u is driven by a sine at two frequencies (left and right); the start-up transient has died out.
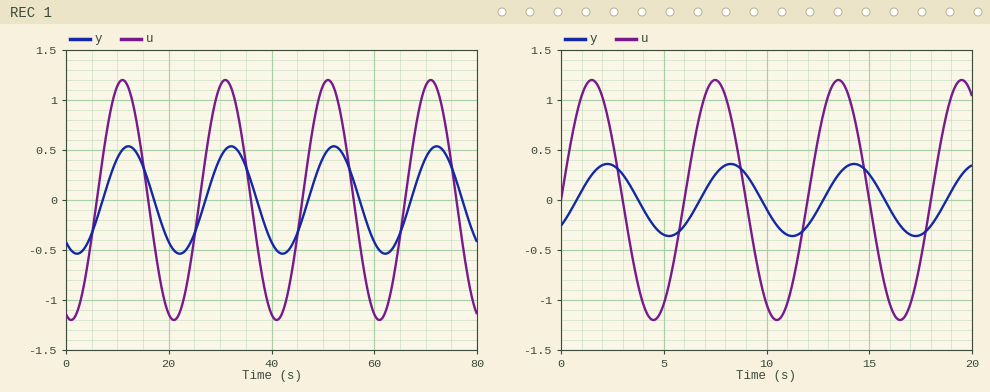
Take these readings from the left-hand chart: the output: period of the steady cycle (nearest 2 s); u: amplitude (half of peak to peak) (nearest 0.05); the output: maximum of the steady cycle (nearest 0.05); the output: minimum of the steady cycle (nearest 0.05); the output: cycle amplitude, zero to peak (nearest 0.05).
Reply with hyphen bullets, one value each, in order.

- 20 s
- 1.20
- 0.55
- -0.55
- 0.55
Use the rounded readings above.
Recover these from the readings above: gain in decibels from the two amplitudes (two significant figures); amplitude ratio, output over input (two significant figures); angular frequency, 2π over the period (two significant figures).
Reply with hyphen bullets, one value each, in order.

- -6.8 dB
- 0.46
- 0.31 rad/s
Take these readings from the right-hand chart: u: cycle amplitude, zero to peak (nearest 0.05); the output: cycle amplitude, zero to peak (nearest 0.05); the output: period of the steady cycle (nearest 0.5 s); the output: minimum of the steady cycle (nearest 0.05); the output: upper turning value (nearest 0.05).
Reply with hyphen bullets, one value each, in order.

- 1.20
- 0.35
- 6.0 s
- -0.35
- 0.35
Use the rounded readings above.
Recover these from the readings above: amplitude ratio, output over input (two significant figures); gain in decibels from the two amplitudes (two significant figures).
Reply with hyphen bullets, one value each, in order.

- 0.29
- -11 dB
